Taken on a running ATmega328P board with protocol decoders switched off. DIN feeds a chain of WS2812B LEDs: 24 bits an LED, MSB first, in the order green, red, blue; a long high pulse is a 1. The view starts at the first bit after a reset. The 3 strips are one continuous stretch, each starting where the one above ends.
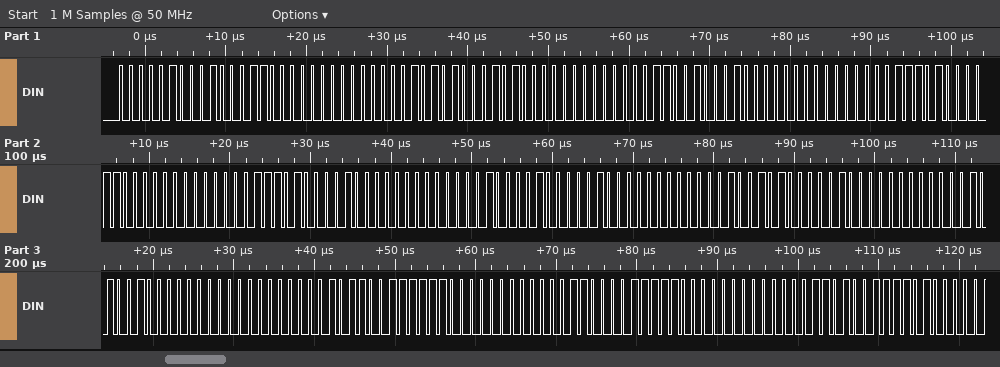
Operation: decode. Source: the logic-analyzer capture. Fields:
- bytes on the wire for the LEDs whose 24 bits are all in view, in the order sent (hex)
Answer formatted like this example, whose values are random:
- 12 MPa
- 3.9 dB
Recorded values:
- 04 46 00 05 45 00 06 44 00 07 43 00 07 42 00 08 41 00 09 41 00 0A 40 00 0B 3F 00 0C 3E 00
